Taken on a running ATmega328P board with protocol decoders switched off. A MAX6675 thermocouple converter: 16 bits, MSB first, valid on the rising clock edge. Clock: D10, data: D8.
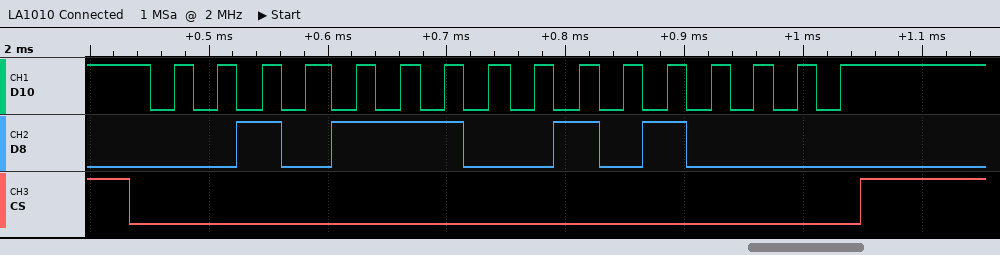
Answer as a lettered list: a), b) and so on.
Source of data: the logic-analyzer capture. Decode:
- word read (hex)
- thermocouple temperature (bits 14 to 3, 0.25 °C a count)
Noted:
a) 0x2E50
b) 370.50 °C
